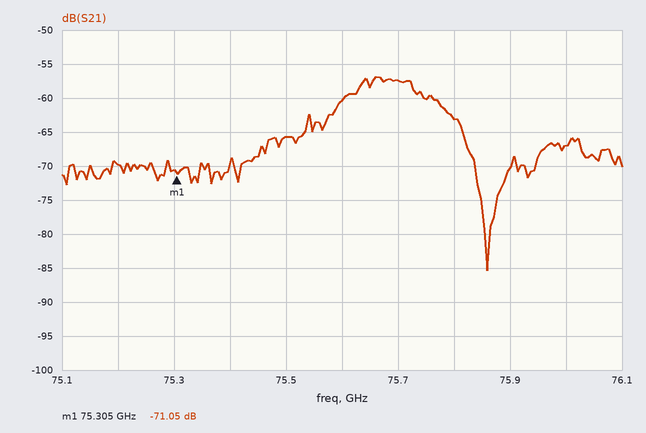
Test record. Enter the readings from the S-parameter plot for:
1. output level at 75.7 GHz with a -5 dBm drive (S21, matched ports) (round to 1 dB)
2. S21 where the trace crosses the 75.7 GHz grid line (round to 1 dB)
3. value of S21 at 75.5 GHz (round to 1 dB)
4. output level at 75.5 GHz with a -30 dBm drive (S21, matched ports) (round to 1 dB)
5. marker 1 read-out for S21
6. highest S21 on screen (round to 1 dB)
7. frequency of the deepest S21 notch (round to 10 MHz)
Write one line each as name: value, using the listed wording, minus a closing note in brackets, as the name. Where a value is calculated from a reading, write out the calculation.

output level at 75.7 GHz with a -5 dBm drive (S21, matched ports): -5 dBm + (-57 dB) = -62 dBm
S21 where the trace crosses the 75.7 GHz grid line: -57 dB
value of S21 at 75.5 GHz: -66 dB
output level at 75.5 GHz with a -30 dBm drive (S21, matched ports): -30 dBm + (-66 dB) = -96 dBm
marker 1 read-out for S21: -71.05 dB
highest S21 on screen: -57 dB
frequency of the deepest S21 notch: 75.86 GHz
